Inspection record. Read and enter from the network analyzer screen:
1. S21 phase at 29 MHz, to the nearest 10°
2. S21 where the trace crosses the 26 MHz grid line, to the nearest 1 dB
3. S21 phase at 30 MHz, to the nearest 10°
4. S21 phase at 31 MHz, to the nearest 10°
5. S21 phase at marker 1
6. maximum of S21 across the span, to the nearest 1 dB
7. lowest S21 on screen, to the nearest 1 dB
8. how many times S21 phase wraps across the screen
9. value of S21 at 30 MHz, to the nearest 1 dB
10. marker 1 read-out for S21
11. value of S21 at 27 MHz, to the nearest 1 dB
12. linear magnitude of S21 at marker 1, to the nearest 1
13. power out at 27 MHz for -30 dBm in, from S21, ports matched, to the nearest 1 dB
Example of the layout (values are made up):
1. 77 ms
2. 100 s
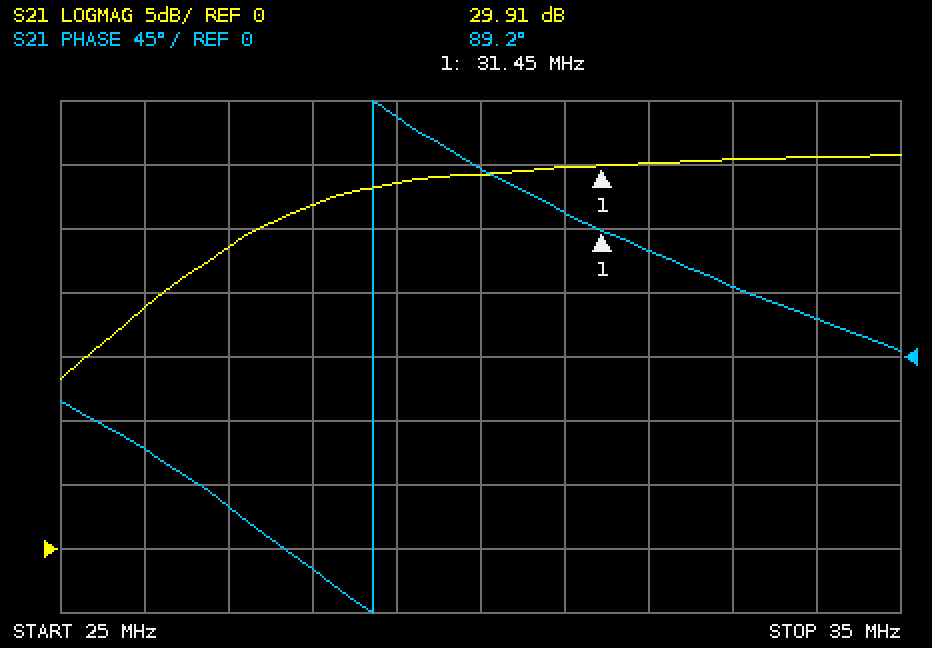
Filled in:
1. 170°
2. 19 dB
3. 130°
4. 100°
5. 89.2°
6. 31 dB
7. 13 dB
8. 1
9. 29 dB
10. 29.91 dB
11. 24 dB
12. 31
13. -6 dBm
